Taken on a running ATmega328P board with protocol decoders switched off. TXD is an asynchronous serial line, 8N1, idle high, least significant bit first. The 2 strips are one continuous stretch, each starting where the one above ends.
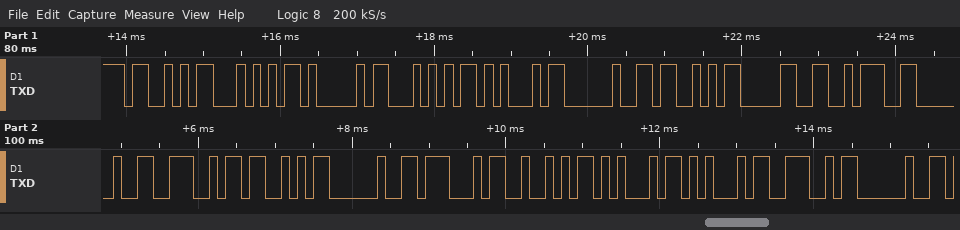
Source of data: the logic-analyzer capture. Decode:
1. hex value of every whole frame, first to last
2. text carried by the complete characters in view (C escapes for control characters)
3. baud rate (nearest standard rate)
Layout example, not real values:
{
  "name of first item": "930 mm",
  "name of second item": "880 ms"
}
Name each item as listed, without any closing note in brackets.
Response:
{
  "hex value of every whole frame, first to last": "53 54 41 54 45 20 53 30 3A 20 4E 53 20 47 52 45 45 4E 20",
  "text carried by the complete characters in view": "\"STATE S0: NS GREEN \"",
  "baud rate": "9600 baud"
}
